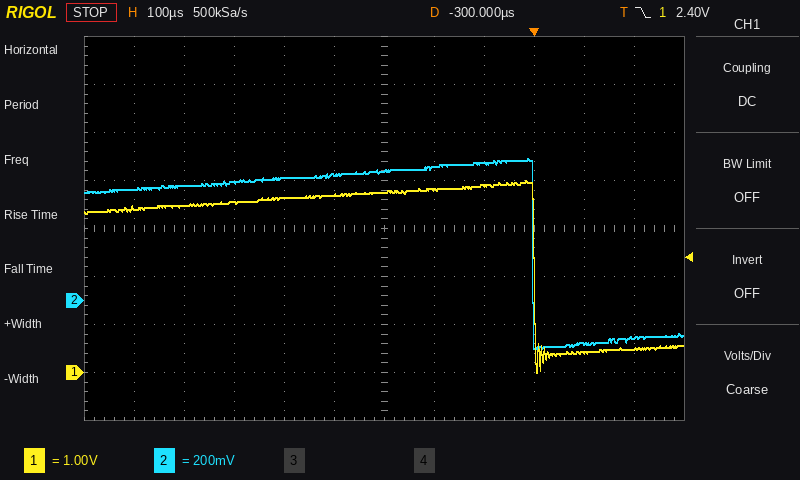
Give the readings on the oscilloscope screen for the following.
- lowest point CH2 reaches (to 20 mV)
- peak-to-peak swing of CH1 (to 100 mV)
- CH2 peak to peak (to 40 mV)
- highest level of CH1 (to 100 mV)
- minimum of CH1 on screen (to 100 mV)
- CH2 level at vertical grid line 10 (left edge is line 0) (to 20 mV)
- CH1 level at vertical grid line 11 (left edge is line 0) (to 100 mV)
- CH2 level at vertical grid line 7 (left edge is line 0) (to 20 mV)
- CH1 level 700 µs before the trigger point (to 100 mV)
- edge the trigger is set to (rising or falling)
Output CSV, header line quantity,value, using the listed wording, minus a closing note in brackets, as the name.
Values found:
quantity,value
lowest point CH2 reaches,-200 mV
peak-to-peak swing of CH1,4.0 V
CH2 peak to peak,800 mV
highest level of CH1,4.0 V
minimum of CH1 on screen,0.0 V
CH2 level at vertical grid line 10 (left edge is line 0),-180 mV
CH1 level at vertical grid line 11 (left edge is line 0),500 mV
CH2 level at vertical grid line 7 (left edge is line 0),560 mV
CH1 level 700 µs before the trigger point,3.5 V
edge the trigger is set to,falling
